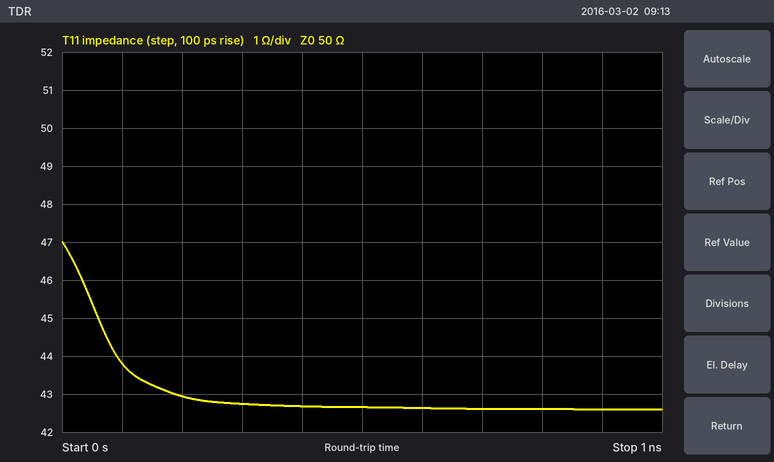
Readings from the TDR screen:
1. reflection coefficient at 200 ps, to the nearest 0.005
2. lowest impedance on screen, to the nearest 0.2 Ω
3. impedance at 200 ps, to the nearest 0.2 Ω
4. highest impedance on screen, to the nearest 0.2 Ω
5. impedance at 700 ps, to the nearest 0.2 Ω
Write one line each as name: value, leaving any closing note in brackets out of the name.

reflection coefficient at 200 ps, to the nearest 0.005: -0.075
lowest impedance on screen, to the nearest 0.2 Ω: 42.6 Ω
impedance at 200 ps, to the nearest 0.2 Ω: 43.0 Ω
highest impedance on screen, to the nearest 0.2 Ω: 47.0 Ω
impedance at 700 ps, to the nearest 0.2 Ω: 42.6 Ω
